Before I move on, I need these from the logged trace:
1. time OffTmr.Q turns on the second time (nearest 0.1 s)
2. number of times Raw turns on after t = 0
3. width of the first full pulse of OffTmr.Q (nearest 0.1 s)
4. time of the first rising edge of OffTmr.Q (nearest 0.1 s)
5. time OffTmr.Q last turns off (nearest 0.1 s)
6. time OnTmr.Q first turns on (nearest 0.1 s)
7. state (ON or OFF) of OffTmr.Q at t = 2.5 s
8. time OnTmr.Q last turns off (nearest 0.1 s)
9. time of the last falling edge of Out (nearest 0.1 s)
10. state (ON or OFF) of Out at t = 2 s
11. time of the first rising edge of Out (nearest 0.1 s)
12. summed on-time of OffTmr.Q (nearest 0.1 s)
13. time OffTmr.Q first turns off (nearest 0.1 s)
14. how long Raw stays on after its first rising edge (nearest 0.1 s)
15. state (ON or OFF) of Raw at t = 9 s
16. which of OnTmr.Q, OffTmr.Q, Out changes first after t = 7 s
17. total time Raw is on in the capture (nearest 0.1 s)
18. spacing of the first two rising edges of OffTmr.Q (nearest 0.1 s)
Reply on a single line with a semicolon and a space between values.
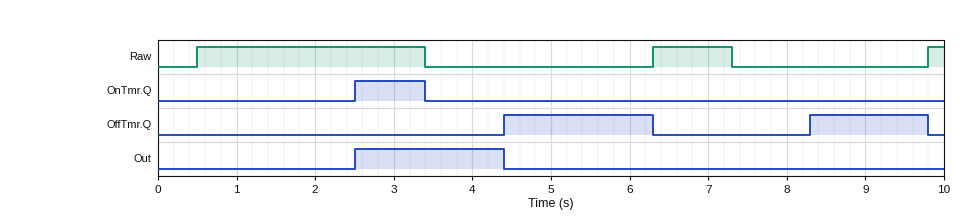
8.3 s; 3; 1.9 s; 4.4 s; 9.8 s; 2.5 s; OFF; 3.4 s; 4.4 s; OFF; 2.5 s; 3.4 s; 6.3 s; 2.9 s; OFF; OffTmr.Q; 4.1 s; 3.9 s
